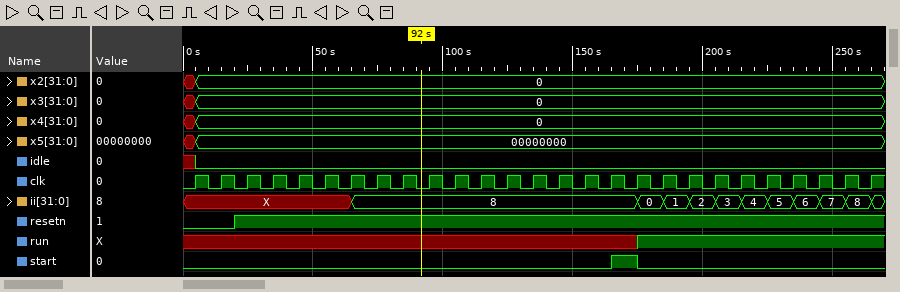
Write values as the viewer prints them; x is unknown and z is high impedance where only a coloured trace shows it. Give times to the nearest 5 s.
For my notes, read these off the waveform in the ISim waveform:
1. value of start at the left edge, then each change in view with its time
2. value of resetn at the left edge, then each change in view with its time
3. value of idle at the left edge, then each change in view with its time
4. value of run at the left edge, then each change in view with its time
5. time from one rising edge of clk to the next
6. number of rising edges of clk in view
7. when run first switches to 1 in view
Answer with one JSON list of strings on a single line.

["0, 1 at 165 s, 0 at 175 s", "0, 1 at 20 s", "x, 0 at 5 s", "x, 1 at 175 s", "10 s", "27", "175 s"]
